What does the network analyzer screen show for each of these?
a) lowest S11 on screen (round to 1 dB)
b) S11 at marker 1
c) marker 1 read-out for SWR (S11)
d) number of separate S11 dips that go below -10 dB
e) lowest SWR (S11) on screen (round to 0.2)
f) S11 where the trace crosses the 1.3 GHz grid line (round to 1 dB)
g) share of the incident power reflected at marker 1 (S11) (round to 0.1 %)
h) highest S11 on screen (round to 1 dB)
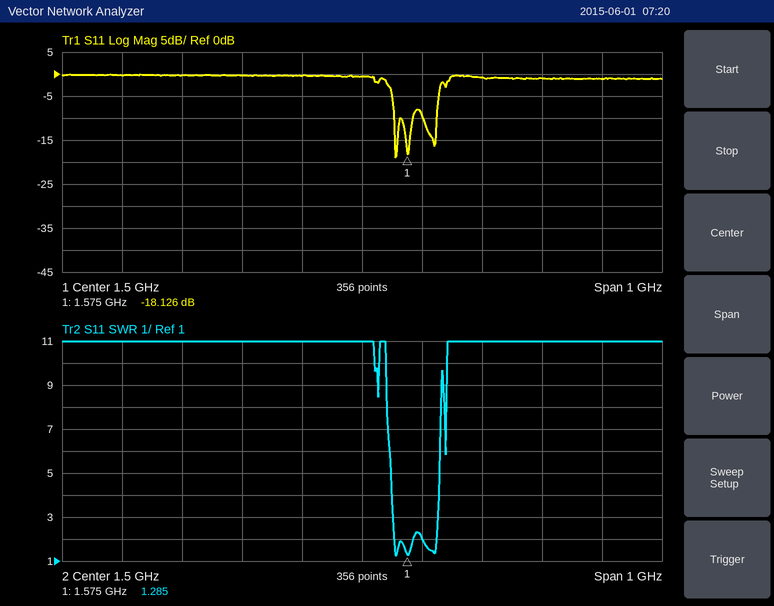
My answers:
-19 dB
-18.126 dB
1.285
3
1.2
0 dB
1.5 %
0 dB
